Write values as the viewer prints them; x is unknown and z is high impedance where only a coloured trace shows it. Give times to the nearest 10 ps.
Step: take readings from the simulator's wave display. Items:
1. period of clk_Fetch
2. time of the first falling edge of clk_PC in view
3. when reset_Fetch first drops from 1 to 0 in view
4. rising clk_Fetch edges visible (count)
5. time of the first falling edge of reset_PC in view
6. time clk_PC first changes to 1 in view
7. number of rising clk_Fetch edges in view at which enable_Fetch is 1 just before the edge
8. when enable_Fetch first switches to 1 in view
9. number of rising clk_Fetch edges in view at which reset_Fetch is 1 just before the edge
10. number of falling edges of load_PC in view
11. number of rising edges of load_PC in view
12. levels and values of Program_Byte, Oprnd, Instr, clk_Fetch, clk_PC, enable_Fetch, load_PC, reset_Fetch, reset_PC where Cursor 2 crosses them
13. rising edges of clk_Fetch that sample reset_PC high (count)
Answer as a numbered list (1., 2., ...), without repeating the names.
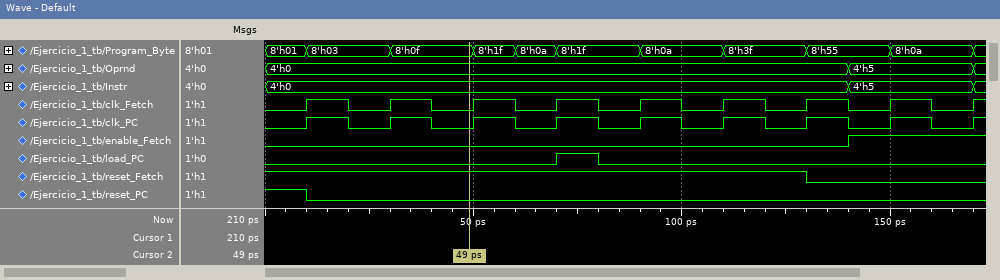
1. 20 ps
2. 20 ps
3. 130 ps
4. 9
5. 10 ps
6. 10 ps
7. 2
8. 140 ps
9. 7
10. 1
11. 1
12. Program_Byte=8'h0f, Oprnd=4'h0, Instr=4'h0, clk_Fetch=0, clk_PC=0, enable_Fetch=0, load_PC=0, reset_Fetch=1, reset_PC=0
13. 1
